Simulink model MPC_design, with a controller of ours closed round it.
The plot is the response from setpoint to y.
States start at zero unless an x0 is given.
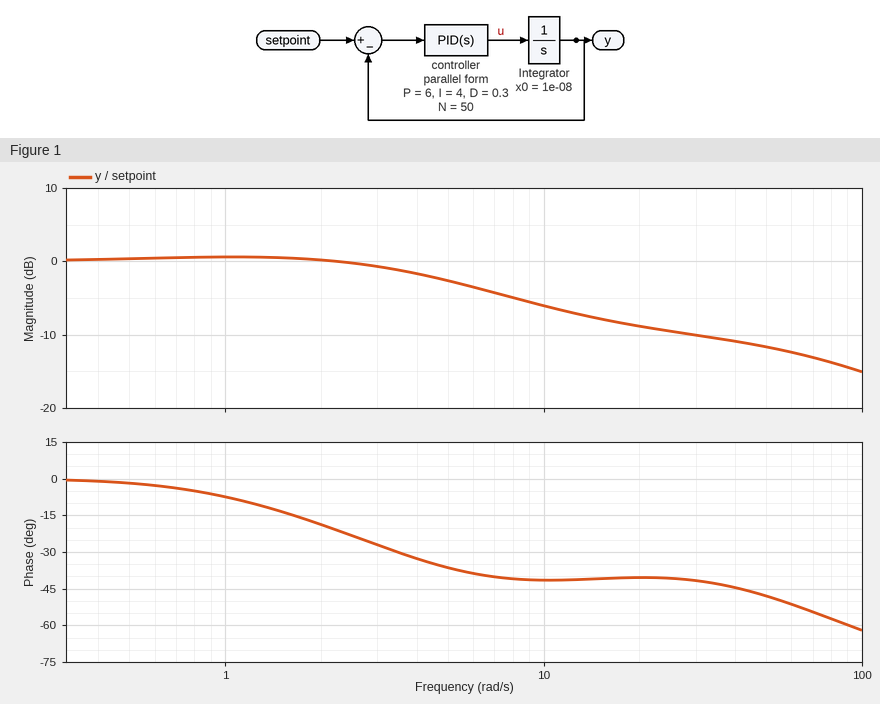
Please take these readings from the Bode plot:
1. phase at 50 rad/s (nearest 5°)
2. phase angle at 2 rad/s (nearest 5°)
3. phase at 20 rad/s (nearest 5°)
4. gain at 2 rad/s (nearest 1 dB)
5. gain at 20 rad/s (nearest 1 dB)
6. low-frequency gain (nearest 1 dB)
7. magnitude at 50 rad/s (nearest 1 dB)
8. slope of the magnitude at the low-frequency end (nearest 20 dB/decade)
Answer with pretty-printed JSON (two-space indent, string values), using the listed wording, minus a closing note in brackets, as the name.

{
  "phase at 50 rad/s": "-50°",
  "phase angle at 2 rad/s": "-20°",
  "phase at 20 rad/s": "-40°",
  "gain at 2 rad/s": "0 dB",
  "gain at 20 rad/s": "-9 dB",
  "low-frequency gain": "0 dB",
  "magnitude at 50 rad/s": "-12 dB",
  "slope of the magnitude at the low-frequency end": "0 dB/decade"
}
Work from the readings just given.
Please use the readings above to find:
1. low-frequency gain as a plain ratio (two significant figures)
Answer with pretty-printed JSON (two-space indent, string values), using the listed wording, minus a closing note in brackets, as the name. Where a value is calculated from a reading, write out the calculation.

{
  "low-frequency gain as a plain ratio": "10^(0 / 20) = 1.0"
}
